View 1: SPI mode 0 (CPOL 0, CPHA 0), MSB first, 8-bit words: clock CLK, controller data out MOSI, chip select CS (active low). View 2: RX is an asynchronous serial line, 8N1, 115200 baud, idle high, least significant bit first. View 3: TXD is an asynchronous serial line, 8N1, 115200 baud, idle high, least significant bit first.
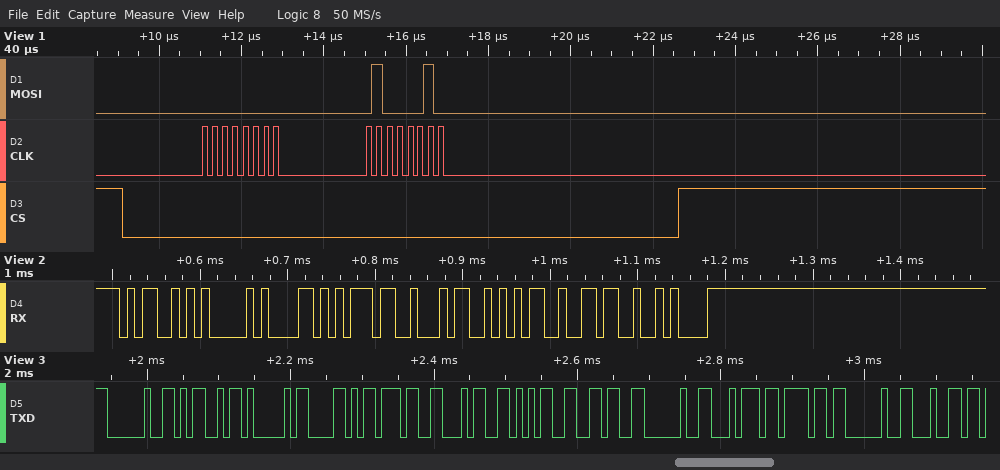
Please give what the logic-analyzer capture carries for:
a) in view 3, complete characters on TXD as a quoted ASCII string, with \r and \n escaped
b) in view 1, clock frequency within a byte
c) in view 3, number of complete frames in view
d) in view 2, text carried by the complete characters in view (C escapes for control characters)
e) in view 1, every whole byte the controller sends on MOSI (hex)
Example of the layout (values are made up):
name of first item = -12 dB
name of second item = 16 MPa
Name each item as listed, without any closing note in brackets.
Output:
in view 3, complete characters on TXD as a quoted ASCII string, with \r and \n escaped = " MAX7456 to d"
in view 1, clock frequency within a byte = 4 MHz
in view 3, number of complete frames in view = 13
in view 2, text carried by the complete characters in view = "MAX7456\n"
in view 1, every whole byte the controller sends on MOSI = 00 42
